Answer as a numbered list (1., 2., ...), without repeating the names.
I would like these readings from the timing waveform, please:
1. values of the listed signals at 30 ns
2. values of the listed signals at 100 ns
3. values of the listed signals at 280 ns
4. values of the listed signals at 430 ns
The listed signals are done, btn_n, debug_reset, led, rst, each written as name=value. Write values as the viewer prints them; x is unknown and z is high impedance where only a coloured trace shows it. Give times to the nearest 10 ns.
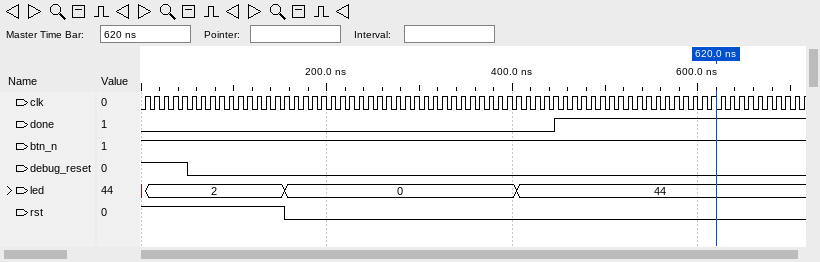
1. done=0, btn_n=1, debug_reset=1, led=2, rst=1
2. done=0, btn_n=1, debug_reset=0, led=2, rst=1
3. done=0, btn_n=1, debug_reset=0, led=0, rst=0
4. done=0, btn_n=1, debug_reset=0, led=44, rst=0
